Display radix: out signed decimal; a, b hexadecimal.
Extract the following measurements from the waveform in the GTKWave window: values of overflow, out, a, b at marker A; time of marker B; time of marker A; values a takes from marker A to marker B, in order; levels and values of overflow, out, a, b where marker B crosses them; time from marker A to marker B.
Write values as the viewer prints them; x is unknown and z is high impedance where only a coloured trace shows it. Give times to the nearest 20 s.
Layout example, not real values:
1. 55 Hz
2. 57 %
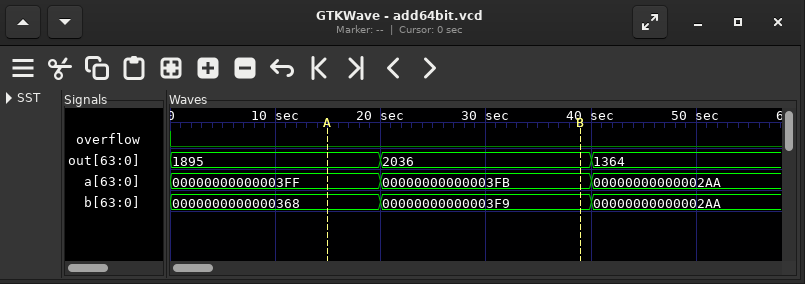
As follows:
1. overflow=0, out=1895, a=00000000000003FF, b=0000000000000368
2. 40 s
3. 20 s
4. 00000000000003FF, 00000000000003FB
5. overflow=0, out=2036, a=00000000000003FB, b=00000000000003F9
6. 20 s
